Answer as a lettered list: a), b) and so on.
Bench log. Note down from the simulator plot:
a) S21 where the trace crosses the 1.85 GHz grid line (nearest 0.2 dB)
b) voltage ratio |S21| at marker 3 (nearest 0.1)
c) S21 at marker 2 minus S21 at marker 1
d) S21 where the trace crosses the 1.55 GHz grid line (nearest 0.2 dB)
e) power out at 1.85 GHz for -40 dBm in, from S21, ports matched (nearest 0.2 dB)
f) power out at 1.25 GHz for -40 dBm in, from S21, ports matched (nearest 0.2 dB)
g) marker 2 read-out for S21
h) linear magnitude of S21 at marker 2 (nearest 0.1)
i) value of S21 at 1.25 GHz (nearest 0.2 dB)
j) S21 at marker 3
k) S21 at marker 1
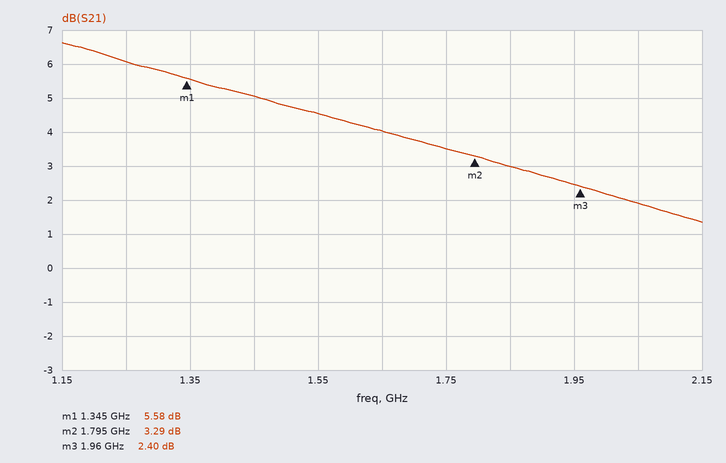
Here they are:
a) 3.0 dB
b) 1.3
c) -2.29 dB
d) 4.6 dB
e) -37.0 dBm
f) -34.0 dBm
g) 3.29 dB
h) 1.5
i) 6.0 dB
j) 2.40 dB
k) 5.58 dB
